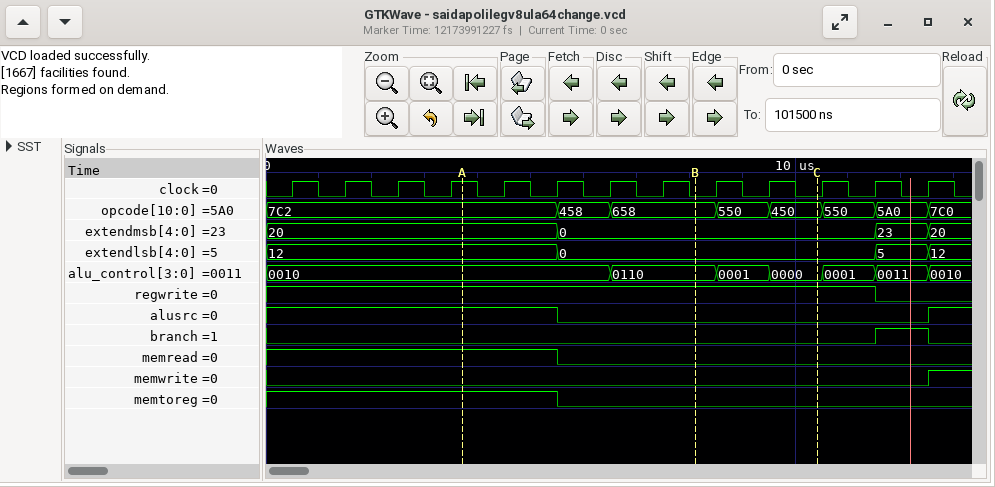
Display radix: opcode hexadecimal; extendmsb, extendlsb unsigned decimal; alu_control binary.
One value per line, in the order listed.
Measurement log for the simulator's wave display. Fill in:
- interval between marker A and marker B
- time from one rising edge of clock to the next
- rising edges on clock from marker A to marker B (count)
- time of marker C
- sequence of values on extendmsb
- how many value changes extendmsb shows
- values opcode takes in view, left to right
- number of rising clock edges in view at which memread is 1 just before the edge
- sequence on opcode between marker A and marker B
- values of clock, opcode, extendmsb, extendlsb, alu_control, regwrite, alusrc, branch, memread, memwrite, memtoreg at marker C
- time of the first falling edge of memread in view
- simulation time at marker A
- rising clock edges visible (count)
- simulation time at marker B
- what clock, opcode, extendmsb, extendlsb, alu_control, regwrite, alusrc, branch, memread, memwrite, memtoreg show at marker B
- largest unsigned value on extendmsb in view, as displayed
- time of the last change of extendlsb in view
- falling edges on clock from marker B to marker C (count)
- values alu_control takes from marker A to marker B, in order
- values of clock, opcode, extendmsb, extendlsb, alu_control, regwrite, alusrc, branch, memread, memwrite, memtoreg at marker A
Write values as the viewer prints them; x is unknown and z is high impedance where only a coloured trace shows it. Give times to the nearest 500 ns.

4500 ns
1000 ns
4
10500 ns
20, 0, 23, 20
3
7C2, 458, 658, 550, 450, 550, 5A0, 7C0
6
7C2, 458, 658
clock=0, opcode=450, extendmsb=0, extendlsb=0, alu_control=0000, regwrite=1, alusrc=0, branch=0, memread=0, memwrite=0, memtoreg=0
5500 ns
3500 ns
13
8000 ns
clock=0, opcode=658, extendmsb=0, extendlsb=0, alu_control=0110, regwrite=1, alusrc=0, branch=0, memread=0, memwrite=0, memtoreg=0
23
12500 ns
2
0010, 0110
clock=1, opcode=7C2, extendmsb=20, extendlsb=12, alu_control=0010, regwrite=1, alusrc=1, branch=0, memread=1, memwrite=0, memtoreg=1
